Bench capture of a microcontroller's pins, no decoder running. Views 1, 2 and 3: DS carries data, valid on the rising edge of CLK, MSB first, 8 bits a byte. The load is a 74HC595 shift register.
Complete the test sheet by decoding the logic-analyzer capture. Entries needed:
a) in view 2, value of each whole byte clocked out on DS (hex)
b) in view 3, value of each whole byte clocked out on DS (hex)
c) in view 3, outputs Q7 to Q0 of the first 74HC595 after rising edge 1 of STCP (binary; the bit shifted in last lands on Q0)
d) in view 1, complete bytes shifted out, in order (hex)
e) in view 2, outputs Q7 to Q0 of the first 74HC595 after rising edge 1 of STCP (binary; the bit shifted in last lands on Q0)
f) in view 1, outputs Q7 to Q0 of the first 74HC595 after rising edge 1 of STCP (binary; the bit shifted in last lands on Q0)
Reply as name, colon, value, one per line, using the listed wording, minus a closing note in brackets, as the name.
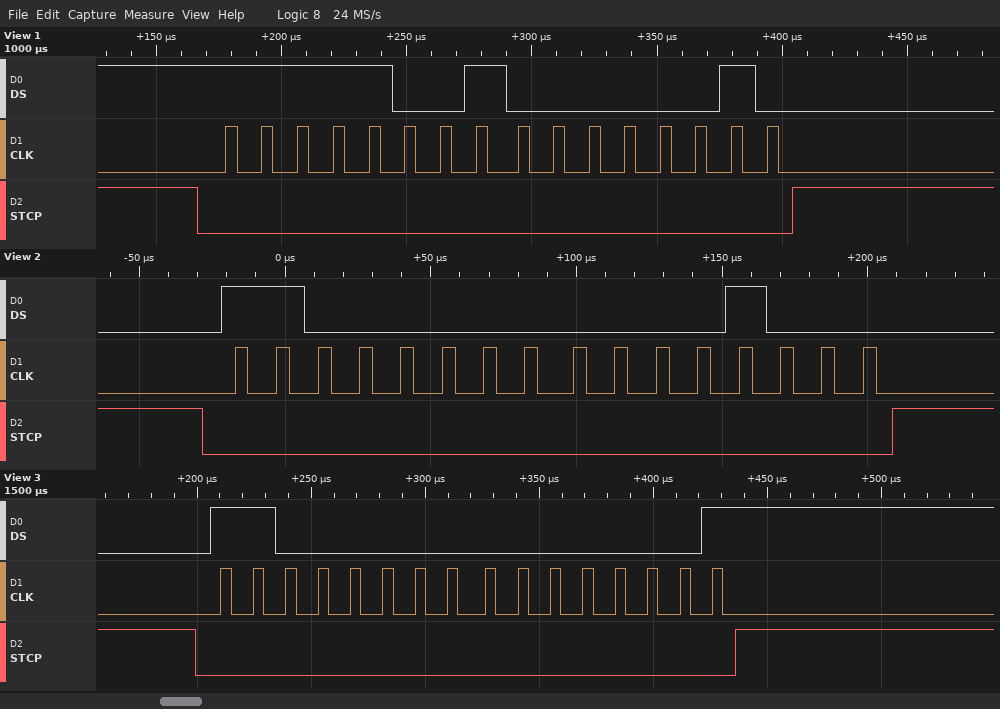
in view 2, value of each whole byte clocked out on DS: 0xC0 0x08
in view 3, value of each whole byte clocked out on DS: 0xC0 0x01
in view 3, outputs Q7 to Q0 of the first 74HC595 after rising edge 1 of STCP: 00000001
in view 1, complete bytes shifted out, in order: F9 02
in view 2, outputs Q7 to Q0 of the first 74HC595 after rising edge 1 of STCP: 00001000
in view 1, outputs Q7 to Q0 of the first 74HC595 after rising edge 1 of STCP: 00000010
